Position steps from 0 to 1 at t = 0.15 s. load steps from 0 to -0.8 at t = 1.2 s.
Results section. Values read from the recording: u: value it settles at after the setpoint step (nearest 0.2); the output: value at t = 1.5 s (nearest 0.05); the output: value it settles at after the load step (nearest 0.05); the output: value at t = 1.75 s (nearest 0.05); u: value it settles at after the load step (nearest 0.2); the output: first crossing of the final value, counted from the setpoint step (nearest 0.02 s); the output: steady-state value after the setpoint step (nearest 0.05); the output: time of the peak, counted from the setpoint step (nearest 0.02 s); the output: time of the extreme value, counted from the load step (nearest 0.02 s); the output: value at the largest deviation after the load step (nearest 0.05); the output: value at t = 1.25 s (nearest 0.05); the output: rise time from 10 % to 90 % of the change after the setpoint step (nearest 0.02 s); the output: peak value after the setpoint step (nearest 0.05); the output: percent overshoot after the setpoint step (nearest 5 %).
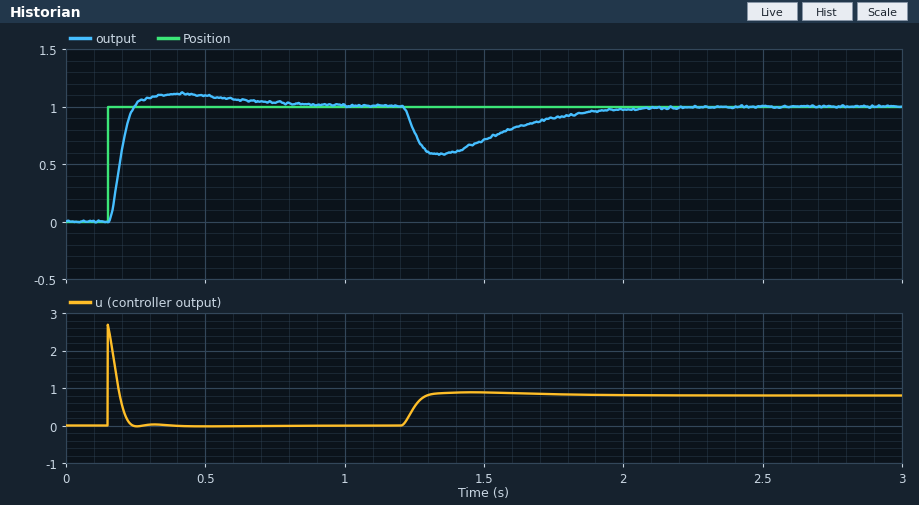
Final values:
0.0
0.70
1.00
0.90
0.8
0.10 s
1.00
0.26 s
0.14 s
0.60
0.80
0.06 s
1.10
10 %
